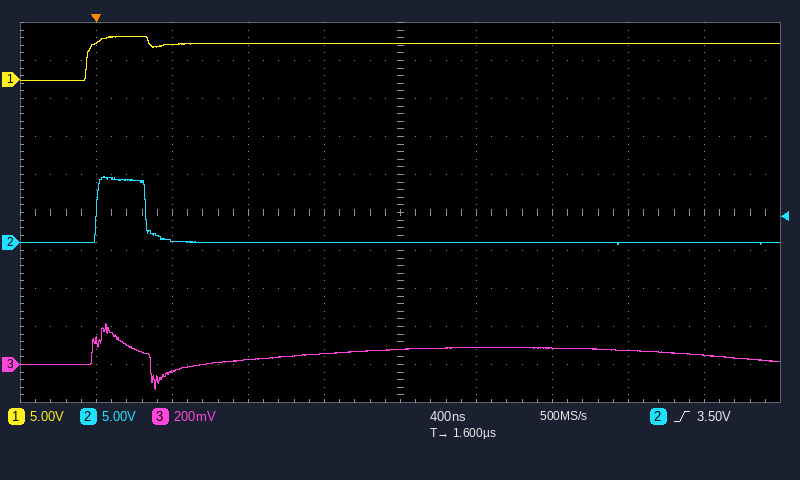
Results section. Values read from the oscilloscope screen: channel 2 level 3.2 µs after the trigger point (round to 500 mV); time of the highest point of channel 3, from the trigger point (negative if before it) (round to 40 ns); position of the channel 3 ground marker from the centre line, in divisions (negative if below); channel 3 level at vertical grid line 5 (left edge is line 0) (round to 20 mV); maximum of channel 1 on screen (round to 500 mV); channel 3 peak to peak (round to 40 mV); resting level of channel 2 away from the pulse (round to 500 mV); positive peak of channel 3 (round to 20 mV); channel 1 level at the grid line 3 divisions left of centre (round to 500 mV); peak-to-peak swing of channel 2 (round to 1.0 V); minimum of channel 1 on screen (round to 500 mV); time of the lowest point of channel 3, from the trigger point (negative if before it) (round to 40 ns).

0.0 V
+40 ns
-4.0 div
80 mV
5.5 V
360 mV
0.0 V
220 mV
4.5 V
9.0 V
0.0 V
+320 ns
